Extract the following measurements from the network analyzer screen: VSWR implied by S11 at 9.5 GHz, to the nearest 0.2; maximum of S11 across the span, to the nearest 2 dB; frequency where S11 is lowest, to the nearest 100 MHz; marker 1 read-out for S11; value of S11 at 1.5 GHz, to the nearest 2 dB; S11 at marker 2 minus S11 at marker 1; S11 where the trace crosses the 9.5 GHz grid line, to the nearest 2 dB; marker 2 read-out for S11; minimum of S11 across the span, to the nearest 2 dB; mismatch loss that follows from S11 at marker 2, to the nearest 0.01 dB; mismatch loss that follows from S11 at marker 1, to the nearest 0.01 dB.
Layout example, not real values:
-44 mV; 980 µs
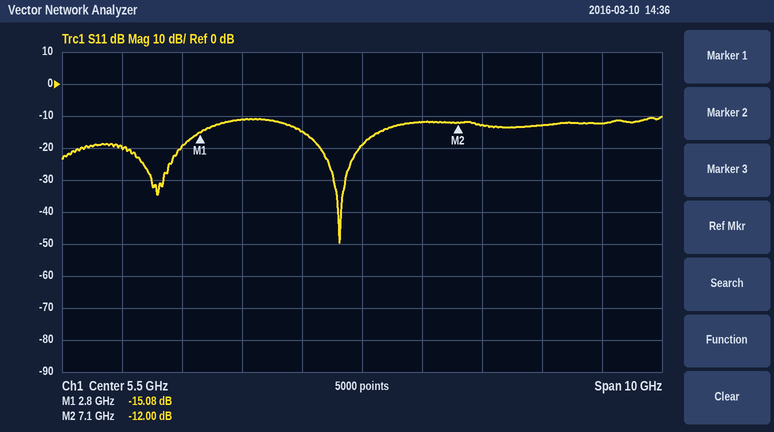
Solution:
1.6; -10 dB; 5.1 GHz; -15.08 dB; -20 dB; 3.08 dB; -12 dB; -12.00 dB; -50 dB; 0.28 dB; 0.14 dB
